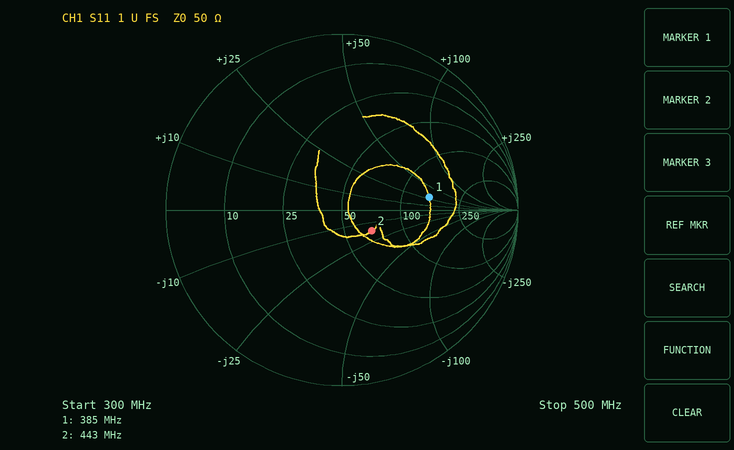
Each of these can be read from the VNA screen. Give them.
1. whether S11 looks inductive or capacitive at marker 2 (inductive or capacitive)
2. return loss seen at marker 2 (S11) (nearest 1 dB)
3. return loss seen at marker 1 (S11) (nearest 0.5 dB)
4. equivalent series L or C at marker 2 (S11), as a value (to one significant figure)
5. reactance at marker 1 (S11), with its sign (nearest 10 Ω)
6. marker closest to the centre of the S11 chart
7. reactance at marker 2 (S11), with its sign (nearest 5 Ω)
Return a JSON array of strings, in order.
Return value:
["capacitive", "14 dB", "6.0 dB", "20 pF", "+30 Ω", "marker 2", "-15 Ω"]
